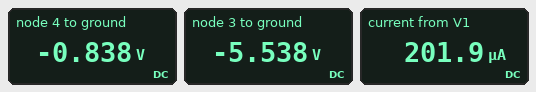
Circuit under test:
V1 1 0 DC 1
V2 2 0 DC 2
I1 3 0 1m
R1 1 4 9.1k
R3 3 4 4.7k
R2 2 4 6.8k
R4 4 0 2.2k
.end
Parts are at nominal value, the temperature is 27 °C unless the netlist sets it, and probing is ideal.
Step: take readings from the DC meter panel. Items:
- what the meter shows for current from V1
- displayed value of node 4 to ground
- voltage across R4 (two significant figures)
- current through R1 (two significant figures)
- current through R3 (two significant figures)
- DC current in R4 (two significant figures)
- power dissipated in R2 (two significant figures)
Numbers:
201.9 µA
-0.838 V
840 mV
200 µA
1.0 mA
380 µA
1.2 mW
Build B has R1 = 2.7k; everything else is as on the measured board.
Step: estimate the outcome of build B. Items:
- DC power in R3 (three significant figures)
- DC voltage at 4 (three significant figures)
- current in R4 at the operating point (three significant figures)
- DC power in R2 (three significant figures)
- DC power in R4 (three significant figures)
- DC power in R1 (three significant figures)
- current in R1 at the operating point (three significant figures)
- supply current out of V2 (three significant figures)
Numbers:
4.70 mW
-345 mV
157 µA
809 µW
54.2 µW
670 µW
498 µA
345 µA
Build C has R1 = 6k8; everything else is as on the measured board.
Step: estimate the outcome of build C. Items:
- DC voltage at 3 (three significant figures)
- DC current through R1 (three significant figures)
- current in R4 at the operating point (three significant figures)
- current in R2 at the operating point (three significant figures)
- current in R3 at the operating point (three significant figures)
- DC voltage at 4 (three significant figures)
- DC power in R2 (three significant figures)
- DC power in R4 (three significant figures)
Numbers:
-5.45 V
257 µA
339 µA
404 µA
1.00 mA
-746 mV
1.11 mW
253 µW
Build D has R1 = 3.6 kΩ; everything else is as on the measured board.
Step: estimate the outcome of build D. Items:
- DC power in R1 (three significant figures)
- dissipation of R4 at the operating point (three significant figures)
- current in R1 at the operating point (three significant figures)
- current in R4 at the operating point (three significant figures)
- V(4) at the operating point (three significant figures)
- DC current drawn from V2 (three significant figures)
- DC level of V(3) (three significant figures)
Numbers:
614 µW
108 µW
413 µA
221 µA
-487 mV
366 µA
-5.19 V
